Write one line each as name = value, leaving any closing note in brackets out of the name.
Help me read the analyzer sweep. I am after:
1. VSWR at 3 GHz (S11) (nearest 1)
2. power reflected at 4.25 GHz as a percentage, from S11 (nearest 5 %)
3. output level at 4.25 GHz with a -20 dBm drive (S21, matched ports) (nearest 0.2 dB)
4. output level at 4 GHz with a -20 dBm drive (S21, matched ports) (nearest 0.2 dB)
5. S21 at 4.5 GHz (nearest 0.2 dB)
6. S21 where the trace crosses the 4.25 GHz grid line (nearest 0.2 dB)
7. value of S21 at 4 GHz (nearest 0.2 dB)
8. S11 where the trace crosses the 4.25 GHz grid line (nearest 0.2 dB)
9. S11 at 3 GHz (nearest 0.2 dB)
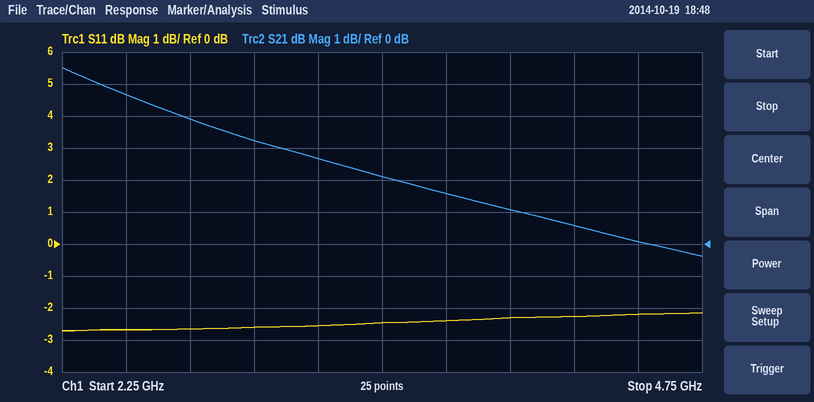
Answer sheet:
VSWR at 3 GHz (S11) = 7
power reflected at 4.25 GHz as a percentage, from S11 = 60 %
output level at 4.25 GHz with a -20 dBm drive (S21, matched ports) = -19.4 dBm
output level at 4 GHz with a -20 dBm drive (S21, matched ports) = -19.0 dBm
S21 at 4.5 GHz = 0.0 dB
S21 where the trace crosses the 4.25 GHz grid line = 0.6 dB
value of S21 at 4 GHz = 1.0 dB
S11 where the trace crosses the 4.25 GHz grid line = -2.2 dB
S11 at 3 GHz = -2.6 dB
